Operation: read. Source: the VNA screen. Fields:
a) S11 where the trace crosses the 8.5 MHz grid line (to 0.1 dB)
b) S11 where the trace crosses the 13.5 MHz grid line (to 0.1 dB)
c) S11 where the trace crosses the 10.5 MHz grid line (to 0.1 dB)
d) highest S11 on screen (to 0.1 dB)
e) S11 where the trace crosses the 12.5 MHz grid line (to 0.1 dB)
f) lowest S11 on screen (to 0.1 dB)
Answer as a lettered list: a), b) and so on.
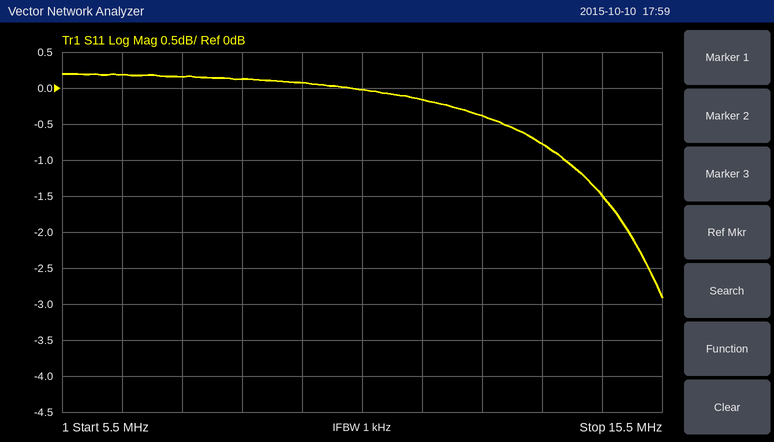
a) 0.1 dB
b) -0.8 dB
c) 0.0 dB
d) 0.2 dB
e) -0.4 dB
f) -2.9 dB
